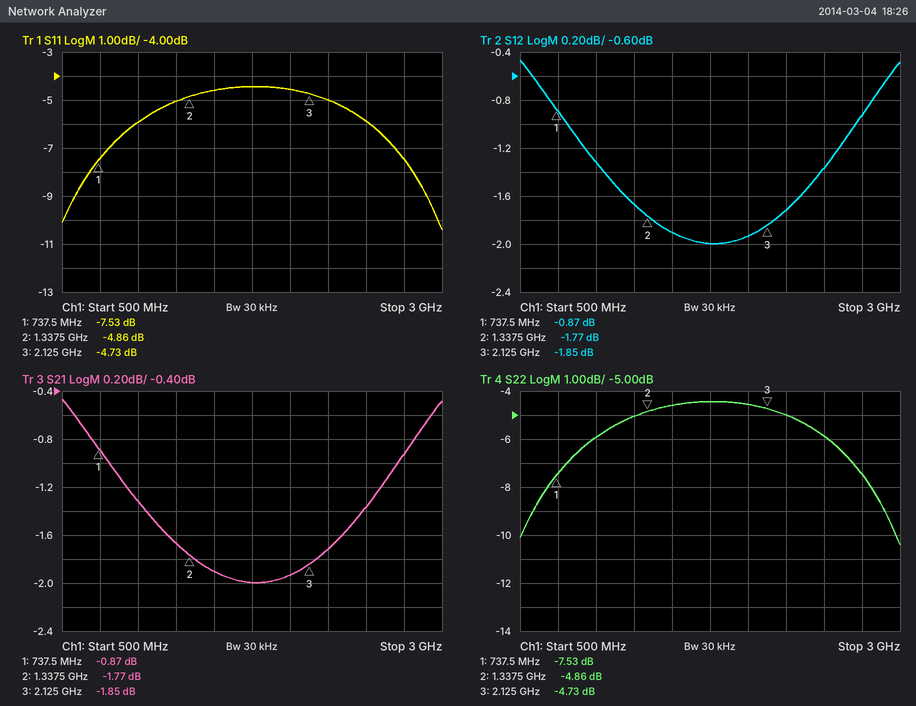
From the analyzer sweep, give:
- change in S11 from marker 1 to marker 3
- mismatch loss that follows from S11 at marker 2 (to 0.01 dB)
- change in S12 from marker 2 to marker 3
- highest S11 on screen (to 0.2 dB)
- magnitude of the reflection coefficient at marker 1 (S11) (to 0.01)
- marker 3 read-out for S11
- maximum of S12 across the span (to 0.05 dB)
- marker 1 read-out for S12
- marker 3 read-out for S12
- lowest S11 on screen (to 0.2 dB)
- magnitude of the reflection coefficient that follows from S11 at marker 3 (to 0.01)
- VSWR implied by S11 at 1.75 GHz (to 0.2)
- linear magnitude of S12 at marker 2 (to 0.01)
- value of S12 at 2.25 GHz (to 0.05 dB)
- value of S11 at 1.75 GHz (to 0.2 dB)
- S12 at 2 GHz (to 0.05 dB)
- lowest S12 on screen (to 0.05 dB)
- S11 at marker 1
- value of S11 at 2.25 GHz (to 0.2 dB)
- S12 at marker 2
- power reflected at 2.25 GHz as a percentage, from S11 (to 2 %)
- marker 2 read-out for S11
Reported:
2.80 dB
1.72 dB
-0.08 dB
-4.4 dB
0.42
-4.73 dB
-0.45 dB
-0.87 dB
-1.85 dB
-10.4 dB
0.58
4.0
0.82
-1.70 dB
-4.4 dB
-1.95 dB
-2.00 dB
-7.53 dB
-5.0 dB
-1.77 dB
32 %
-4.86 dB
